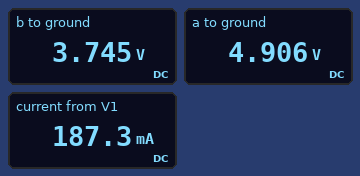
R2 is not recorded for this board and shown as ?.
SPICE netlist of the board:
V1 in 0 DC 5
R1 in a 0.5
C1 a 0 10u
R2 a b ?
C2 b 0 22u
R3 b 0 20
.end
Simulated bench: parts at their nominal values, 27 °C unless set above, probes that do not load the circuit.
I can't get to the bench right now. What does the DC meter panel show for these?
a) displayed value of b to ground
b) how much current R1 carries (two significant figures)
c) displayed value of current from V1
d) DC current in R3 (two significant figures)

3.745 V
190 mA
187.3 mA
190 mA
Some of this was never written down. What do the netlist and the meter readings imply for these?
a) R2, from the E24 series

6.2 Ω
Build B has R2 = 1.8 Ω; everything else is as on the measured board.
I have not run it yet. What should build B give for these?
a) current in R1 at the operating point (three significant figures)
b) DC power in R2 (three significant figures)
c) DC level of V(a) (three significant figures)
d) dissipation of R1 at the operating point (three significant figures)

224 mA
90.5 mW
4.89 V
25.1 mW
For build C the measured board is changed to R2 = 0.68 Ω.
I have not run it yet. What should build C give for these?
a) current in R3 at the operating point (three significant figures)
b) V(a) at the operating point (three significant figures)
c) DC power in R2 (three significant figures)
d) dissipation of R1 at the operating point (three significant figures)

236 mA
4.88 V
37.9 mW
27.9 mW
